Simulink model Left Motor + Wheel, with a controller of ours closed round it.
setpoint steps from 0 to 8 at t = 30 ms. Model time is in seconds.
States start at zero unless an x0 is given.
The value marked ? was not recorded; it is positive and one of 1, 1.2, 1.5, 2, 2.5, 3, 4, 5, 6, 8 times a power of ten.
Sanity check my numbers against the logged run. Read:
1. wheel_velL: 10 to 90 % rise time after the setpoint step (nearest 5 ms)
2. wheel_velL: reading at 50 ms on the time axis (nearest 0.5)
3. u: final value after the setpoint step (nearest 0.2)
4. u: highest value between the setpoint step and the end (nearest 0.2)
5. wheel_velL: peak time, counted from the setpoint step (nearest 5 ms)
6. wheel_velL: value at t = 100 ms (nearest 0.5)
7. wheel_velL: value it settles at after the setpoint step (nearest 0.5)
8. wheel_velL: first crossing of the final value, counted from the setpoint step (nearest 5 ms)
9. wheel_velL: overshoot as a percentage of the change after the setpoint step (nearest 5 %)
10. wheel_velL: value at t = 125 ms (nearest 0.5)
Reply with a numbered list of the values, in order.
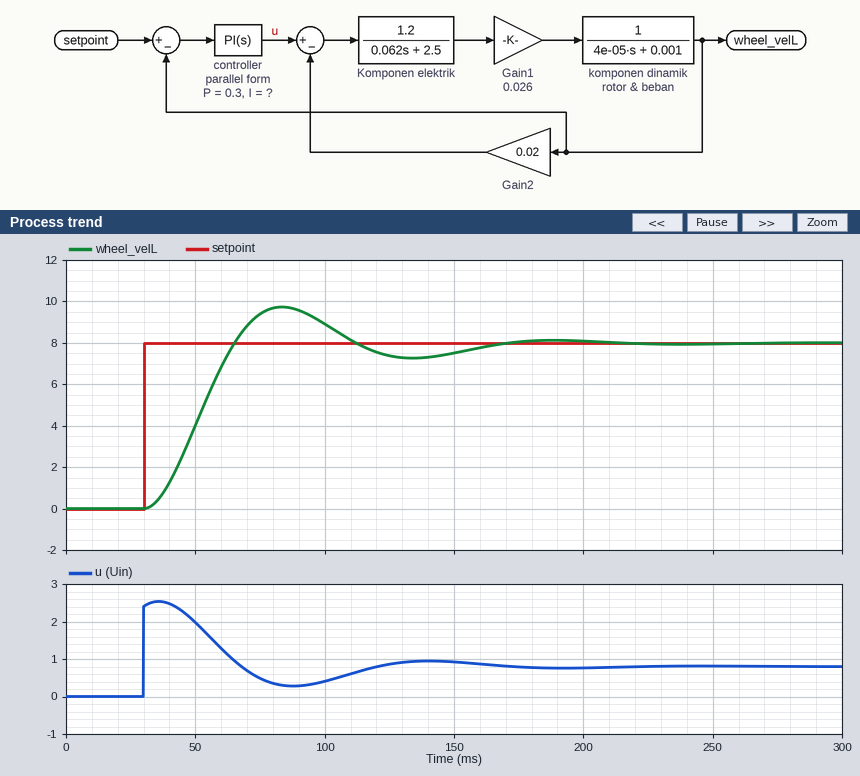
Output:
1. 25 ms
2. 4.0
3. 0.8
4. 2.6
5. 55 ms
6. 9.0
7. 8.0
8. 35 ms
9. 20 %
10. 7.5
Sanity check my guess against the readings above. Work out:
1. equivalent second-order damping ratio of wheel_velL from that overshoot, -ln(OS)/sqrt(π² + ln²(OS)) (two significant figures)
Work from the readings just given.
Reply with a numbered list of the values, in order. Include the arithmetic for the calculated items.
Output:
1. ln(0.2) = -1.609; 1.609 / sqrt(9.870 + 2.590) = 0.46
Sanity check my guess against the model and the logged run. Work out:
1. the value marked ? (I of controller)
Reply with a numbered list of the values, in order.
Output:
1. 6
